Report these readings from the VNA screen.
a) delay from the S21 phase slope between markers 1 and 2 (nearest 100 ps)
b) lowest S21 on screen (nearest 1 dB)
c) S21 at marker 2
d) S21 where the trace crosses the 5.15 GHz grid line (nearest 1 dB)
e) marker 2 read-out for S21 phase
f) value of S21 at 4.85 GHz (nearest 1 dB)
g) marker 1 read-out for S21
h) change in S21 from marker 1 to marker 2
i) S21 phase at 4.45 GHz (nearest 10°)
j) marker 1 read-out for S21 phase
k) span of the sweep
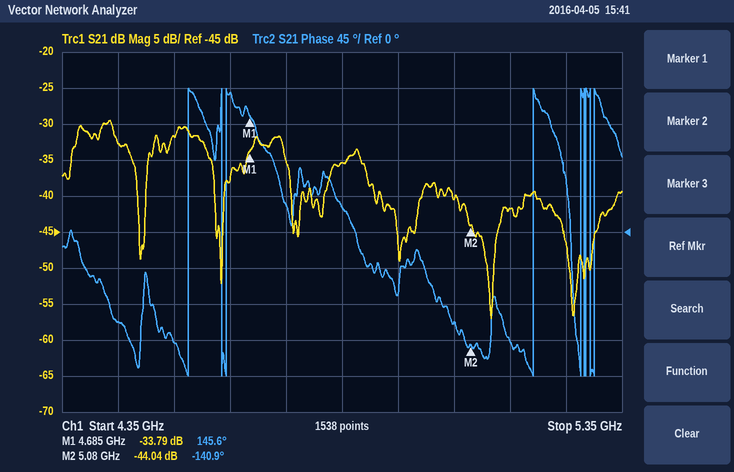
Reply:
2.0 ns
-57 dB
-44.04 dB
-42 dB
-140.9°
-35 dB
-33.79 dB
-10.25 dB
-110°
145.6°
1 GHz
